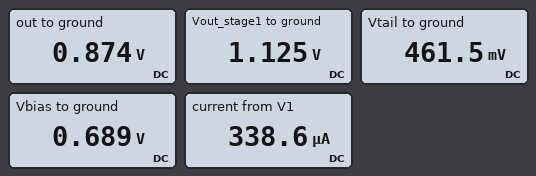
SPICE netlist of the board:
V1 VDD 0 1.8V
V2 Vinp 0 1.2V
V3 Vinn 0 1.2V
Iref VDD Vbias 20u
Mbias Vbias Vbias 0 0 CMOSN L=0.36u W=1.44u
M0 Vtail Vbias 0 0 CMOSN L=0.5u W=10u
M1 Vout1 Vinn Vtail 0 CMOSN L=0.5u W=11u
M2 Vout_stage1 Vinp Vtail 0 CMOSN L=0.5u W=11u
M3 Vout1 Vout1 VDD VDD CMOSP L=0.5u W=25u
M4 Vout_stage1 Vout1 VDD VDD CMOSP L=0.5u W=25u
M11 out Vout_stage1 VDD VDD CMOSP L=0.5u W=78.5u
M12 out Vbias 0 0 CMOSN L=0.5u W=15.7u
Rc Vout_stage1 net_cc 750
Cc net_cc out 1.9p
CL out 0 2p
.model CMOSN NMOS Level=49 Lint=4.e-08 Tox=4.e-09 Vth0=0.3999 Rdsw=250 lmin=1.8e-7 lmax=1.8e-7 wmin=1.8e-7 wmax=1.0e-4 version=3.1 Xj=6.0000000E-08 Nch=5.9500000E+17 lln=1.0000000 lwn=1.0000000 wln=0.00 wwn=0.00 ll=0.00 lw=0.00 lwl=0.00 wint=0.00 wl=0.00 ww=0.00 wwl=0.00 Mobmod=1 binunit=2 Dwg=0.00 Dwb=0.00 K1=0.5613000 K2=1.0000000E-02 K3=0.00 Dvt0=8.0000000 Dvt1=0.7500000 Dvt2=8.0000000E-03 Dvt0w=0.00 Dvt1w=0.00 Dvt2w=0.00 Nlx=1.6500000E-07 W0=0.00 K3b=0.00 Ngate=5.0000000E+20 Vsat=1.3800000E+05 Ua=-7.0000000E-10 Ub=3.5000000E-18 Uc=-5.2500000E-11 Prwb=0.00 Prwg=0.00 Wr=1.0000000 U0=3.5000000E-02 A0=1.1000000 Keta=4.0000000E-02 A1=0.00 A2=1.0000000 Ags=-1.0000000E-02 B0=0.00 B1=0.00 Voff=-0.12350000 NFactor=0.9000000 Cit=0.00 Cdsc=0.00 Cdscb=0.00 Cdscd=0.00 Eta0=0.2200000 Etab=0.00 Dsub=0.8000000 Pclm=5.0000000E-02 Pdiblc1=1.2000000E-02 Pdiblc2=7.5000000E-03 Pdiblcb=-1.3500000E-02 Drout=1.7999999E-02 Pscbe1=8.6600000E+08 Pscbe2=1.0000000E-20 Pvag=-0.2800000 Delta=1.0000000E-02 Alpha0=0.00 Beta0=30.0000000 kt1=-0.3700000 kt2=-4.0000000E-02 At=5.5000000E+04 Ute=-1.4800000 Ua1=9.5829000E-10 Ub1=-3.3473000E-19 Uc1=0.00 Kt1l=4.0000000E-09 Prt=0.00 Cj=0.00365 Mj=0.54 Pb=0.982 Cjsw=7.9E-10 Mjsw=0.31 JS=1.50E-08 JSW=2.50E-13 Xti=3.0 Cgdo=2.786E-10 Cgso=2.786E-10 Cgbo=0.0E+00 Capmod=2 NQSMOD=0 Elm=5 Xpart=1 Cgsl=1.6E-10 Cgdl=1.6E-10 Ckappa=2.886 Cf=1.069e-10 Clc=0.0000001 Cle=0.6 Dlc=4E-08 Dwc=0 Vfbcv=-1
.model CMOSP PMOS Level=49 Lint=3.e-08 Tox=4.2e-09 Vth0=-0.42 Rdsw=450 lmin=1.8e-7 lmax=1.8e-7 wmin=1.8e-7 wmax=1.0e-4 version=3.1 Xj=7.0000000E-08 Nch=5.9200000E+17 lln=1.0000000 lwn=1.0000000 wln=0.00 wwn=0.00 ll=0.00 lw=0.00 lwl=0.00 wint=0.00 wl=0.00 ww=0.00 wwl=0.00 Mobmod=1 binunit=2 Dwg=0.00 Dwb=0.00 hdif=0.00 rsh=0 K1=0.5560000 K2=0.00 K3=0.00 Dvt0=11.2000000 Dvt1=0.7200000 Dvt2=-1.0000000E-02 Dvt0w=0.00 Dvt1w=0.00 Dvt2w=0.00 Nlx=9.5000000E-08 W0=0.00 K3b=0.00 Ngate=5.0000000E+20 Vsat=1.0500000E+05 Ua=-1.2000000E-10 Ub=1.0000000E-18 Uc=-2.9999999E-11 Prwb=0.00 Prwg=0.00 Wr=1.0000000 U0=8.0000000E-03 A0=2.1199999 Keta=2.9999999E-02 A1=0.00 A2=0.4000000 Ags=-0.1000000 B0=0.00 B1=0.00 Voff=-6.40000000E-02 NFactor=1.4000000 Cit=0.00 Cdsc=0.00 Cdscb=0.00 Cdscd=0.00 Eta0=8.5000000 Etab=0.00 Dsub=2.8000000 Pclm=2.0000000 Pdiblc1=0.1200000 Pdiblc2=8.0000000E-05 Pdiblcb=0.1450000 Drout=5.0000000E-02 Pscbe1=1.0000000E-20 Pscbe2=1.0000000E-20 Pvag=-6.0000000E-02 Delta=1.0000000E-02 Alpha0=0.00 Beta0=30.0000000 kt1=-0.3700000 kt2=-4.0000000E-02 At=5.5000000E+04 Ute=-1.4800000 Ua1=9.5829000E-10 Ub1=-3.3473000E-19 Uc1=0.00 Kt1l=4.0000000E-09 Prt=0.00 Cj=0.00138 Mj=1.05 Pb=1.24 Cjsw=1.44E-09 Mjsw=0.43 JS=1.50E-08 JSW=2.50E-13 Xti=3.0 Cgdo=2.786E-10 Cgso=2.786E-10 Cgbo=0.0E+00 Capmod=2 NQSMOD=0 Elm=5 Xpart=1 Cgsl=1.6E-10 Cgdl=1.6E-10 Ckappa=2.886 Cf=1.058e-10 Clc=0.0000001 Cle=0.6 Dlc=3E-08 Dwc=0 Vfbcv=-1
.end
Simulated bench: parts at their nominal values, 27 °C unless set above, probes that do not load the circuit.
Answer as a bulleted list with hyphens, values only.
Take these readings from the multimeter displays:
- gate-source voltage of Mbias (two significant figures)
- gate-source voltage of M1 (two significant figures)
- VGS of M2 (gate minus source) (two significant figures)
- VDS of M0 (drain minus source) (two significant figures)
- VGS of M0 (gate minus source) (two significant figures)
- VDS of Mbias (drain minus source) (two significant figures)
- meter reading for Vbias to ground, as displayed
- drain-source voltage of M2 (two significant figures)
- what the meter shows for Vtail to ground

- 690 mV
- 740 mV
- 740 mV
- 460 mV
- 690 mV
- 690 mV
- 0.689 V
- 660 mV
- 461.5 mV
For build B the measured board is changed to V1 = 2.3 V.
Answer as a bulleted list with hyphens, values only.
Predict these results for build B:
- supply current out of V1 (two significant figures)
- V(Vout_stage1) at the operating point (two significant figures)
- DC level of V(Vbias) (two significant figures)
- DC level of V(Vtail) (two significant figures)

- 350 µA
- 1.6 V
- 690 mV
- 470 mV
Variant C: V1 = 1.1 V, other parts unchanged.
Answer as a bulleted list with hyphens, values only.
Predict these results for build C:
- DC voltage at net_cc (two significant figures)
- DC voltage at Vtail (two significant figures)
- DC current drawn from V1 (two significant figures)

- 430 mV
- 380 mV
- 320 µA
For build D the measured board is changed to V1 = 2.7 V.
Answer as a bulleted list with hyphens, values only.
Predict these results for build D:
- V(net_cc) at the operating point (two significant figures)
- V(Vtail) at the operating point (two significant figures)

- 2.0 V
- 470 mV
